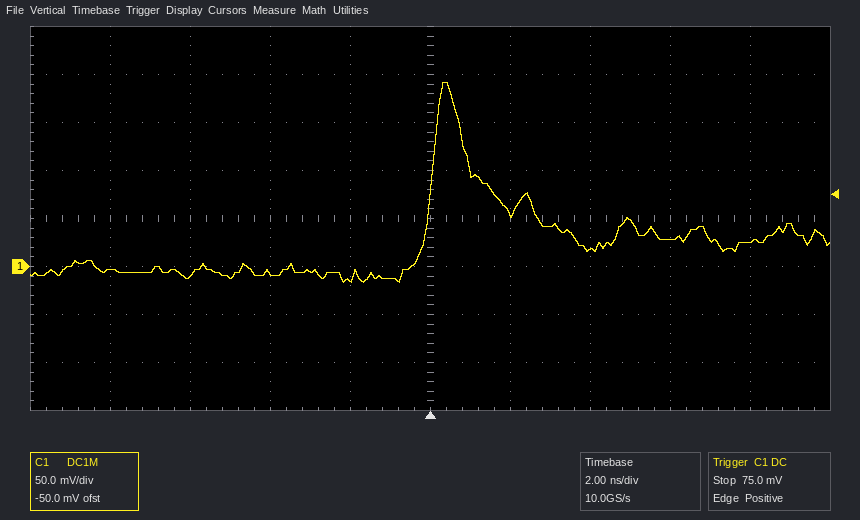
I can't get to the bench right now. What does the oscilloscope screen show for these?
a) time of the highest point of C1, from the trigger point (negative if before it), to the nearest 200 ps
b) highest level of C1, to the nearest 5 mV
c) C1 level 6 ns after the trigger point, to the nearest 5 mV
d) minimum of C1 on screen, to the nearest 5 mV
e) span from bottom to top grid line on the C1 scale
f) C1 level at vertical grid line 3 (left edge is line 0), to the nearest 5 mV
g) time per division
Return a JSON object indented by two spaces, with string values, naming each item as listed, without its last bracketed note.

{
  "time of the highest point of C1, from the trigger point (negative if before it), to the nearest 200 ps": "+400 ps",
  "highest level of C1, to the nearest 5 mV": "190 mV",
  "C1 level 6 ns after the trigger point, to the nearest 5 mV": "30 mV",
  "minimum of C1 on screen, to the nearest 5 mV": "-15 mV",
  "span from bottom to top grid line on the C1 scale": "400 mV",
  "C1 level at vertical grid line 3 (left edge is line 0), to the nearest 5 mV": "-5 mV",
  "time per division": "2 ns"
}
